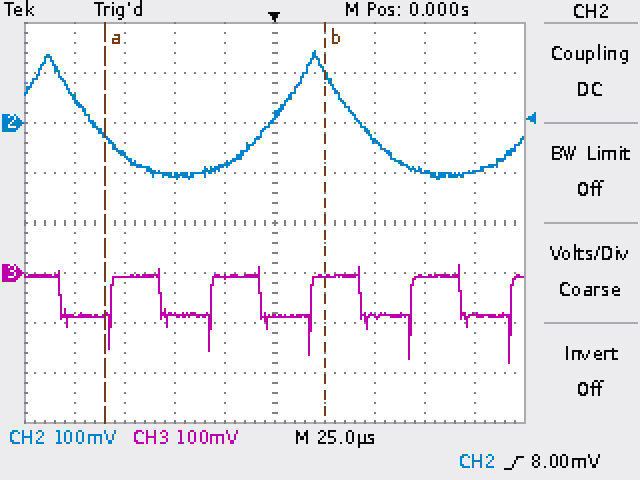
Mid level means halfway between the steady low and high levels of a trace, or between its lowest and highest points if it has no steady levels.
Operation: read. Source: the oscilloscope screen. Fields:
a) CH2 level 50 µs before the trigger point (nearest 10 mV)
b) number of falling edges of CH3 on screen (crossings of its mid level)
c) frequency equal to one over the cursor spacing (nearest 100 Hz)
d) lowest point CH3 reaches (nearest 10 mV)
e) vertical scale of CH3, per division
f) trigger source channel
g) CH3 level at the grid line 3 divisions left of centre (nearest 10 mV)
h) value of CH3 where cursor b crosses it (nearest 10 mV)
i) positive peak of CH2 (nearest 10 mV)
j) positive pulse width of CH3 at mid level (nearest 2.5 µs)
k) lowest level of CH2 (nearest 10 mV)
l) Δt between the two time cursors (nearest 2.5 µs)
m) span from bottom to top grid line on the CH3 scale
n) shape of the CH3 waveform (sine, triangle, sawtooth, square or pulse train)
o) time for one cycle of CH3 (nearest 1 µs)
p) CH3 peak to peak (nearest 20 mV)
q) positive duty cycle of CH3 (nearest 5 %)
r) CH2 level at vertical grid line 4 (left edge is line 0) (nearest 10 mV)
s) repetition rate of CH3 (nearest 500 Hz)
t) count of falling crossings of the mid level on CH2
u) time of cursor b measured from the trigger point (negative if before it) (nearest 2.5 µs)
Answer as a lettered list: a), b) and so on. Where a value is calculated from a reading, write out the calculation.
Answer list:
a) -110 mV
b) 5
c) 1 / 110.0 µs ≈ 9.1 kHz
d) -180 mV
e) 100 mV
f) CH2
g) -10 mV
h) -10 mV
i) 140 mV
j) 25.0 µs
k) -110 mV
l) 110.0 µs
m) 800 mV
n) square
o) 50 µs
p) 200 mV
q) 25.0 µs / 50 µs ≈ 50 %
r) -80 mV
s) 1 / 50 µs ≈ 20.0 kHz
t) 2
u) +25.0 µs
